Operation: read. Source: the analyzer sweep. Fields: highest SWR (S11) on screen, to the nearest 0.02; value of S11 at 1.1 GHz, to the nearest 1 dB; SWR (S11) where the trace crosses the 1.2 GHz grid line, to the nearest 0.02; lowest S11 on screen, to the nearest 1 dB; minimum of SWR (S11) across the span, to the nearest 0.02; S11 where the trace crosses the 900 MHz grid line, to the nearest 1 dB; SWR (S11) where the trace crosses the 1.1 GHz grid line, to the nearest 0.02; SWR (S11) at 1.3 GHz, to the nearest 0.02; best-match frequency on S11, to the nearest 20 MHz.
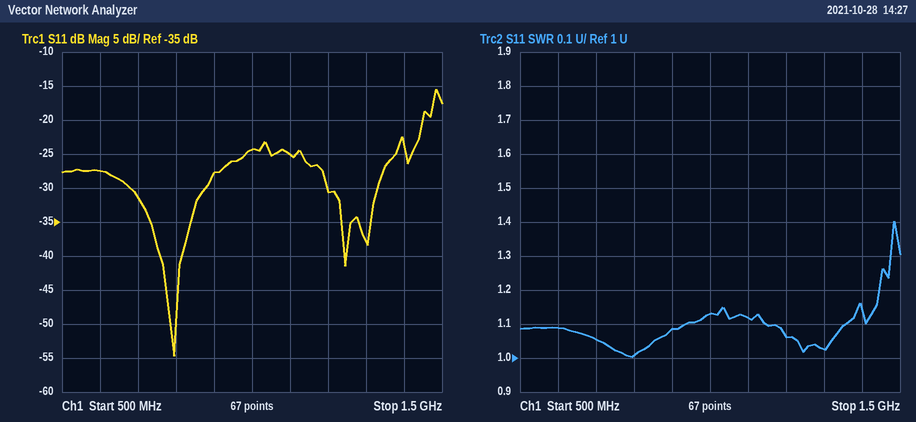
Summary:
1.40
-25 dB
1.06
-55 dB
1.00
-28 dB
1.12
1.02
800 MHz
